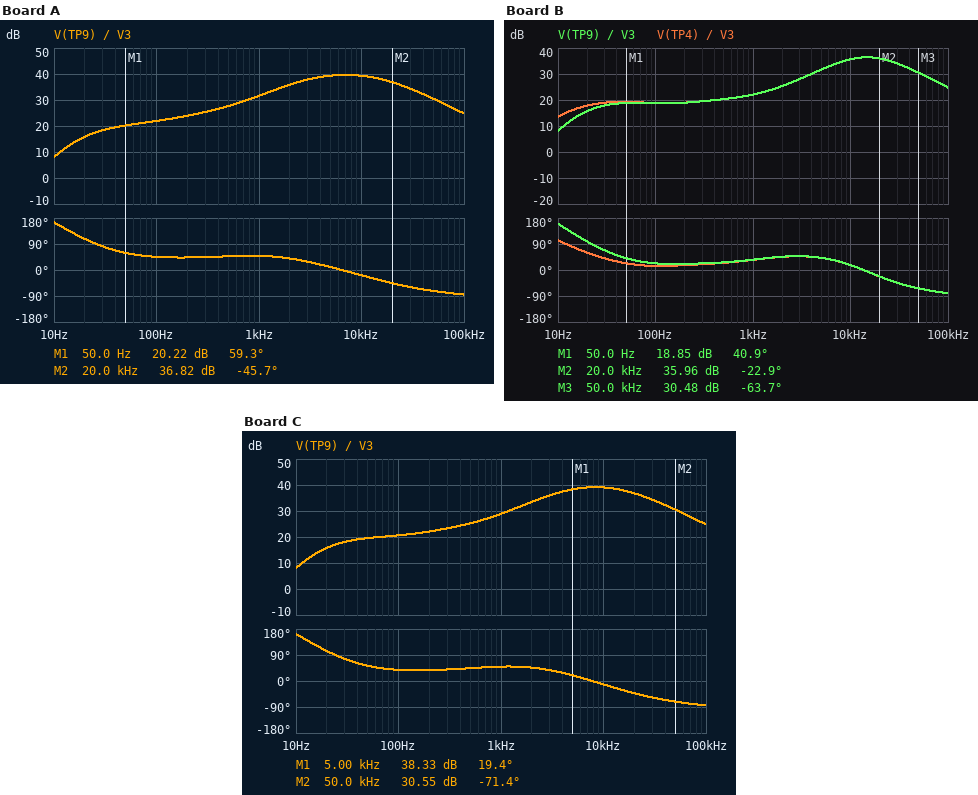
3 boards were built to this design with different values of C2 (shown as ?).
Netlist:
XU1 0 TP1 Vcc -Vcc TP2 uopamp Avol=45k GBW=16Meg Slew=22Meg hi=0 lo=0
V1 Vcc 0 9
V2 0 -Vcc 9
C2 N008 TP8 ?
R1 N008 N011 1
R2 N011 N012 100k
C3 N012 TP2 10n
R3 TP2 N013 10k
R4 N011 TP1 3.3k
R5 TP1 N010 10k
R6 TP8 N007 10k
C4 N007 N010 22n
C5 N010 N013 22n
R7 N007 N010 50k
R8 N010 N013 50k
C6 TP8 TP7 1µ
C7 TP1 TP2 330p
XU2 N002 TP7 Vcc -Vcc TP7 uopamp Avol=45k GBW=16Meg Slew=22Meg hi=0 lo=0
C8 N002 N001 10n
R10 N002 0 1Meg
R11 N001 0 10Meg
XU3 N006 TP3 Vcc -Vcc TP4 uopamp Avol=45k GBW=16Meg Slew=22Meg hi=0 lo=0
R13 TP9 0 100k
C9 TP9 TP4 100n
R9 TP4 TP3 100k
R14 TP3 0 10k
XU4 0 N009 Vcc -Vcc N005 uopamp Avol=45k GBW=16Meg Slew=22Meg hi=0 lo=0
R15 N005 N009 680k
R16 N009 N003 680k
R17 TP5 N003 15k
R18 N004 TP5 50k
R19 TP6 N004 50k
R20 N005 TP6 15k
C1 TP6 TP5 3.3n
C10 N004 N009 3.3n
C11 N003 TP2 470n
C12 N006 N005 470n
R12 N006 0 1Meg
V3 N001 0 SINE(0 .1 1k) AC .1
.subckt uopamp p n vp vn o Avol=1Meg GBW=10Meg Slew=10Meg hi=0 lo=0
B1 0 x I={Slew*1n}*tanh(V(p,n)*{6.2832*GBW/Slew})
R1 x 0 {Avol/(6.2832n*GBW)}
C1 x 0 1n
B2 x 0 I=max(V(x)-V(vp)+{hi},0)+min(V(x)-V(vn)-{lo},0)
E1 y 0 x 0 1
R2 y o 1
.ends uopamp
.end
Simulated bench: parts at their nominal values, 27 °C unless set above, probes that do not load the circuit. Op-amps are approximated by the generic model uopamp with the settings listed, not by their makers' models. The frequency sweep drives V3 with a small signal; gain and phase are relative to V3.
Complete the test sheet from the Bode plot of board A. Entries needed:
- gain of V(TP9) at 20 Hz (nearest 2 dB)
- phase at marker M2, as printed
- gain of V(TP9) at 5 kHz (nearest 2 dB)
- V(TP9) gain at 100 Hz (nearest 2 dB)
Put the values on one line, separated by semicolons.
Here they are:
16 dB; -45.7 deg; 40 dB; 22 dB
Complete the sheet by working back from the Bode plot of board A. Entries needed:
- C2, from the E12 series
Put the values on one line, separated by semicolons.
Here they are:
22 nF
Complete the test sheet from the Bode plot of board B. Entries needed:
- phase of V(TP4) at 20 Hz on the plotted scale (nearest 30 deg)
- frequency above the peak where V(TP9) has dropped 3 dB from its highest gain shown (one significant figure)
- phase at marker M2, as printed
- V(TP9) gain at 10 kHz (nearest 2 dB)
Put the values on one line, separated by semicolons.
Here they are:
60 deg; 30 kHz; -22.9 deg; 36 dB
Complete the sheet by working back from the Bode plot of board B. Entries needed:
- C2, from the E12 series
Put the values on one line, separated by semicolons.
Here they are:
4.7 nF
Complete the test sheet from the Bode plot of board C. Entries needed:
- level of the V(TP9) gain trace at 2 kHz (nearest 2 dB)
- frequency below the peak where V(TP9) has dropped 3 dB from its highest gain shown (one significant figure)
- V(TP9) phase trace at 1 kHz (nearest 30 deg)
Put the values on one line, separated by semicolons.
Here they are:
34 dB; 3 kHz; 60 deg
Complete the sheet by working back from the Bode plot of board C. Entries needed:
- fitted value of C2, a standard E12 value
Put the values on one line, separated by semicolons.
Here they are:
15 nF
